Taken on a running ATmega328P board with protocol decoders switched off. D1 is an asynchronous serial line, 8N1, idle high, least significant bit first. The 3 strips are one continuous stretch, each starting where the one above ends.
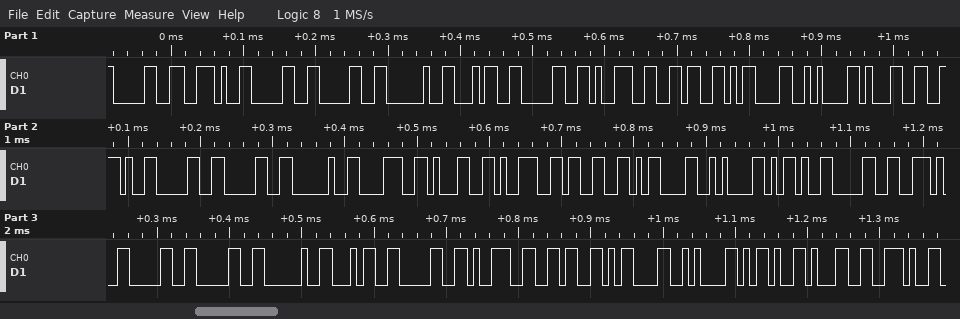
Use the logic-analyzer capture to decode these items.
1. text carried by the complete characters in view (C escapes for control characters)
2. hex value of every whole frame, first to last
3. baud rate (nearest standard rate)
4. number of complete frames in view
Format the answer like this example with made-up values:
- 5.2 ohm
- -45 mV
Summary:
- "0.00 4096\r\n1.00 8193\r\n-0.00 4096\r\n-1."
- 30 2E 30 30 20 34 30 39 36 0D 0A 31 2E 30 30 20 38 31 39 33 0D 0A 2D 30 2E 30 30 20 34 30 39 36 0D 0A 2D 31 2E
- 115200 baud
- 37
